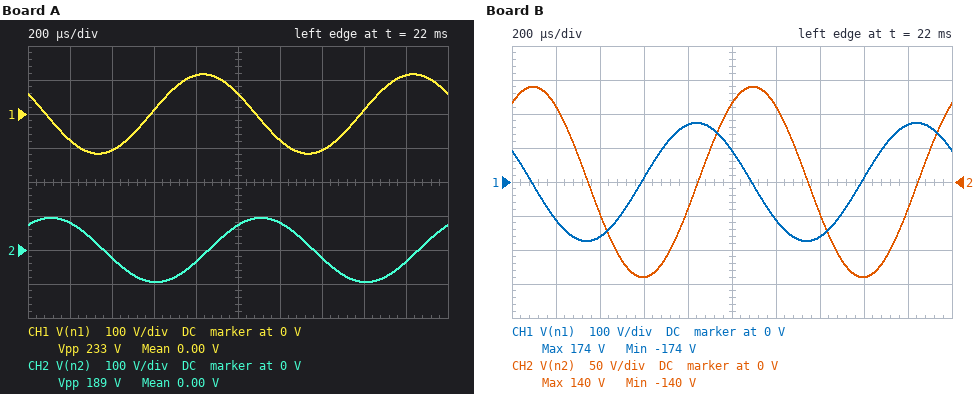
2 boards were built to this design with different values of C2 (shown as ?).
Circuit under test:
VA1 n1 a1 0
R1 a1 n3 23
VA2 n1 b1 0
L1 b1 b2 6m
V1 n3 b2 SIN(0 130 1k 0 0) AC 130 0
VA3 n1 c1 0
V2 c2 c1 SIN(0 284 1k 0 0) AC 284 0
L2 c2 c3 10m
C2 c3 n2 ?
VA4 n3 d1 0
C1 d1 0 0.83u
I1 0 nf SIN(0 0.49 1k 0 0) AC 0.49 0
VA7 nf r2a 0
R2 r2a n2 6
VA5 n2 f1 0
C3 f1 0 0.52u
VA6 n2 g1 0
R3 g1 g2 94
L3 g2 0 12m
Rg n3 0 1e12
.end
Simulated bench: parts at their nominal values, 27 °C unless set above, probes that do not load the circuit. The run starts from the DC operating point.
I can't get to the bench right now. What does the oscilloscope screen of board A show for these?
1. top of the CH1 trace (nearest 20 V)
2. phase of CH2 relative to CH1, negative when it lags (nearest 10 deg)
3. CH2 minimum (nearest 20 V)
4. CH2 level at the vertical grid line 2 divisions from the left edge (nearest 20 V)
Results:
120 V
-100 deg
-100 V
-20 V
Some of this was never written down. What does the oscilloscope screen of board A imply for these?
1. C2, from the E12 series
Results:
390 nF
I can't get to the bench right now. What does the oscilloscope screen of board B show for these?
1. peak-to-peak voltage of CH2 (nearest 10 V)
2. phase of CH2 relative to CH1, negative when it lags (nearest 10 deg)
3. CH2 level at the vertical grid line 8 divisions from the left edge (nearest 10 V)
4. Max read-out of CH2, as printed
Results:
280 V
-90 deg
-140 V
140 V
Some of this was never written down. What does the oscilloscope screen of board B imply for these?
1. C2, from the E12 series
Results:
1 µF
